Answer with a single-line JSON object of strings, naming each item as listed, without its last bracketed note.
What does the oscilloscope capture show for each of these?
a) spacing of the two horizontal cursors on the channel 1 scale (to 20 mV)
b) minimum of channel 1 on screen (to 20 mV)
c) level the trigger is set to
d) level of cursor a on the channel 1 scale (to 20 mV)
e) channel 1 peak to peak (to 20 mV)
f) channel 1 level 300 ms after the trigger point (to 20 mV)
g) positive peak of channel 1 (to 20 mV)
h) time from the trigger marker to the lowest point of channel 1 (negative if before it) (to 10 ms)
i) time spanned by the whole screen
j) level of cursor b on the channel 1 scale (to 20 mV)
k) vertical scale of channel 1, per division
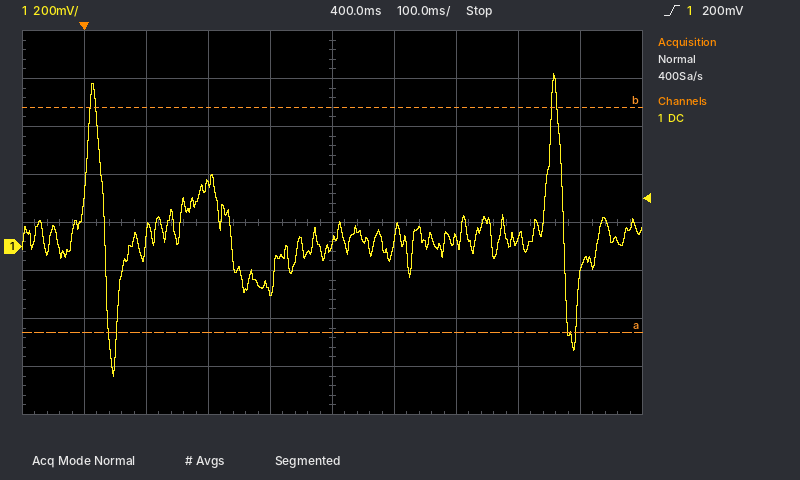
{"spacing of the two horizontal cursors on the channel 1 scale": "940 mV", "minimum of channel 1 on screen": "-540 mV", "level the trigger is set to": "200 mV", "level of cursor a on the channel 1 scale": "-360 mV", "channel 1 peak to peak": "1.26 V", "channel 1 level 300 ms after the trigger point": "-180 mV", "positive peak of channel 1": "720 mV", "time from the trigger marker to the lowest point of channel 1 (negative if before it)": "+50 ms", "time spanned by the whole screen": "1 s", "level of cursor b on the channel 1 scale": "580 mV", "vertical scale of channel 1, per division": "200 mV"}
